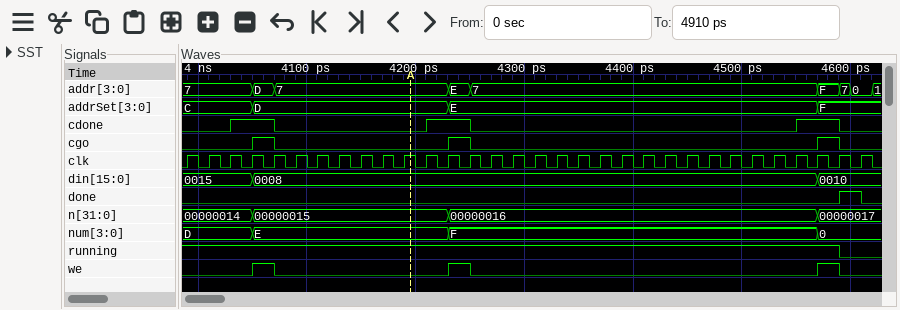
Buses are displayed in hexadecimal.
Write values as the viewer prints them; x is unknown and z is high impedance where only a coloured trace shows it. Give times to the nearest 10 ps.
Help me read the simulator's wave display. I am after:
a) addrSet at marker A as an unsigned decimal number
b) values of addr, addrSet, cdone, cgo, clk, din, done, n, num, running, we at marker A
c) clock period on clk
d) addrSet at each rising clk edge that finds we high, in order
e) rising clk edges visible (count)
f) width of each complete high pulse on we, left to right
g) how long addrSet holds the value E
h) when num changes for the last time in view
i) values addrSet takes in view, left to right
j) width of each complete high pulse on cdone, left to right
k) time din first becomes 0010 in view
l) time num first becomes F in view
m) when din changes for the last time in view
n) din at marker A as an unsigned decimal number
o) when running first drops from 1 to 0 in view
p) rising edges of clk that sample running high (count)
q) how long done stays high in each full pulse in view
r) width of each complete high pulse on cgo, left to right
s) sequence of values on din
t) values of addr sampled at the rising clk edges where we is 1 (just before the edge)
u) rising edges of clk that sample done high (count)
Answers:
13
addr=7, addrSet=D, cdone=0, cgo=0, clk=1, din=0008, done=0, n=00000015, num=E, running=1, we=0
20 ps
D, E, F
32
20 ps, 20 ps, 20 ps
340 ps
4570 ps
C, D, E, F
40 ps, 40 ps, 40 ps
4570 ps
4230 ps
4570 ps
8
4590 ps
31
20 ps
20 ps, 20 ps, 20 ps
0015, 0008, 0010
D, E, F
1
